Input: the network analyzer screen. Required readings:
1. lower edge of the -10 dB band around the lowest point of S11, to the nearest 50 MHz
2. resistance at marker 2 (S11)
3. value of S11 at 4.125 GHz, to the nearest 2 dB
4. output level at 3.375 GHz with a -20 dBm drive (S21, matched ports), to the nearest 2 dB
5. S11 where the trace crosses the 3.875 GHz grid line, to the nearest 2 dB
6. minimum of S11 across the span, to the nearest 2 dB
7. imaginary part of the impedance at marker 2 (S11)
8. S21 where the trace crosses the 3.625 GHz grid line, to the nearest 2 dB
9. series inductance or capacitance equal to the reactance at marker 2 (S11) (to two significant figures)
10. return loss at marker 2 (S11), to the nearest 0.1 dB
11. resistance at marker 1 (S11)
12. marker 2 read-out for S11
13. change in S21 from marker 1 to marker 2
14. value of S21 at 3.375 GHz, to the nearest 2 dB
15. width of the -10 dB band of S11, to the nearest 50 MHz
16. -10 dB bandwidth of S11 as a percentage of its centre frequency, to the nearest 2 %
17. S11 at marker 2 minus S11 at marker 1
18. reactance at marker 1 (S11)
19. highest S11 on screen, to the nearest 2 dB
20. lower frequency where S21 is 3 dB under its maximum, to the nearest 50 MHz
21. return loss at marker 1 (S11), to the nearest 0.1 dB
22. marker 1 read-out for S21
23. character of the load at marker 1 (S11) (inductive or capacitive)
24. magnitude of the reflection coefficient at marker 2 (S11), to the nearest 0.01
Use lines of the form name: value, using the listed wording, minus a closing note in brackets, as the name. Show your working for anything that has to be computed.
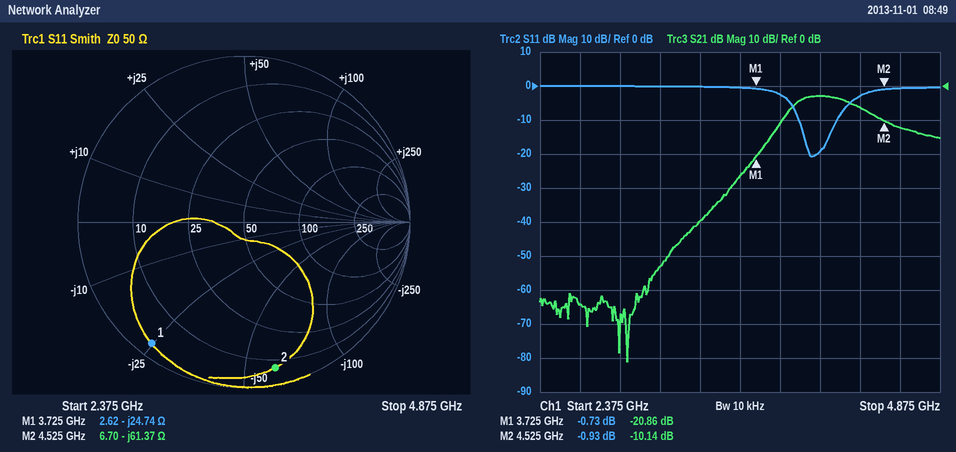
lower edge of the -10 dB band around the lowest point of S11, to the nearest 50 MHz: 4.00 GHz
resistance at marker 2: 6.70 Ω
value of S11 at 4.125 GHz, to the nearest 2 dB: -20 dB
output level at 3.375 GHz with a -20 dBm drive (S21, matched ports), to the nearest 2 dB: -20 dBm + (-40 dB) = -60 dBm
S11 where the trace crosses the 3.875 GHz grid line, to the nearest 2 dB: -2 dB
minimum of S11 across the span, to the nearest 2 dB: -20 dB
imaginary part of the impedance at marker 2: -61.37 Ω
S21 where the trace crosses the 3.625 GHz grid line, to the nearest 2 dB: -26 dB
series inductance or capacitance equal to the reactance at marker 2 (S11): C = 1/(2π × 4.525 GHz × 61.37 Ω) ≈ 573 fF, so 570 fF to two significant figures
return loss at marker 2 (S11), to the nearest 0.1 dB: 0.9 dB
resistance at marker 1: 2.62 Ω
marker 2 read-out for S11: -0.93 dB
change in S21 from marker 1 to marker 2: -10.14 − (-20.86) = 10.72 dB
value of S21 at 3.375 GHz, to the nearest 2 dB: -40 dB
width of the -10 dB band of S11, to the nearest 50 MHz: 4.25 GHz − 4.00 GHz = 250 MHz
-10 dB bandwidth of S11 as a percentage of its centre frequency, to the nearest 2 %: 250 MHz / 4.125 GHz ≈ 6 %
S11 at marker 2 minus S11 at marker 1: -0.93 − (-0.73) = -0.20 dB
reactance at marker 1: -24.74 Ω
highest S11 on screen, to the nearest 2 dB: 0 dB
lower frequency where S21 is 3 dB under its maximum, to the nearest 50 MHz: 3.95 GHz
return loss at marker 1 (S11), to the nearest 0.1 dB: 0.7 dB
marker 1 read-out for S21: -20.86 dB
character of the load at marker 1 (S11): capacitive
magnitude of the reflection coefficient at marker 2 (S11), to the nearest 0.01: 10^(-0.93/20) ≈ 0.90
